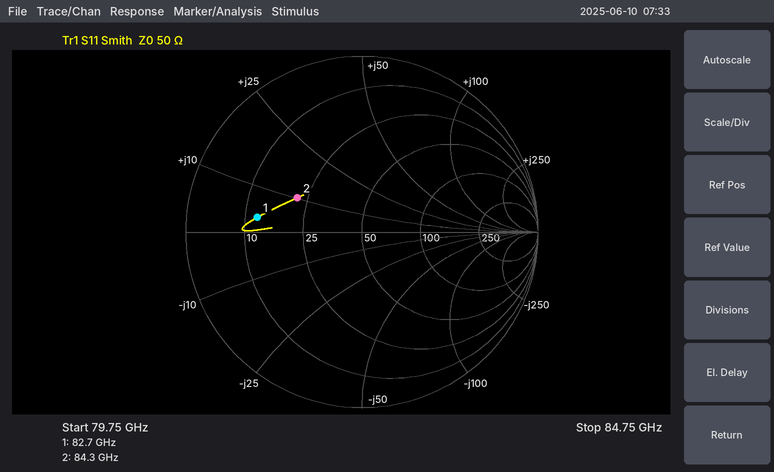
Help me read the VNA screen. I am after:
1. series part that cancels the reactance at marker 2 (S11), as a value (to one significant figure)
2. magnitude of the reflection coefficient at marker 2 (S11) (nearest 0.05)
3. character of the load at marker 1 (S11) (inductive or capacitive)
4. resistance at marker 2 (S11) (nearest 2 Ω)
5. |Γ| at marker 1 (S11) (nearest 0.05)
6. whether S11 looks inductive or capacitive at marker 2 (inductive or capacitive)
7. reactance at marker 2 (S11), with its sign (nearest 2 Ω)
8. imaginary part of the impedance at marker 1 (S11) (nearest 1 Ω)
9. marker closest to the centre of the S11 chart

200 fF
0.40
inductive
22 Ω
0.60
inductive
+10 Ω
+3 Ω
marker 2
